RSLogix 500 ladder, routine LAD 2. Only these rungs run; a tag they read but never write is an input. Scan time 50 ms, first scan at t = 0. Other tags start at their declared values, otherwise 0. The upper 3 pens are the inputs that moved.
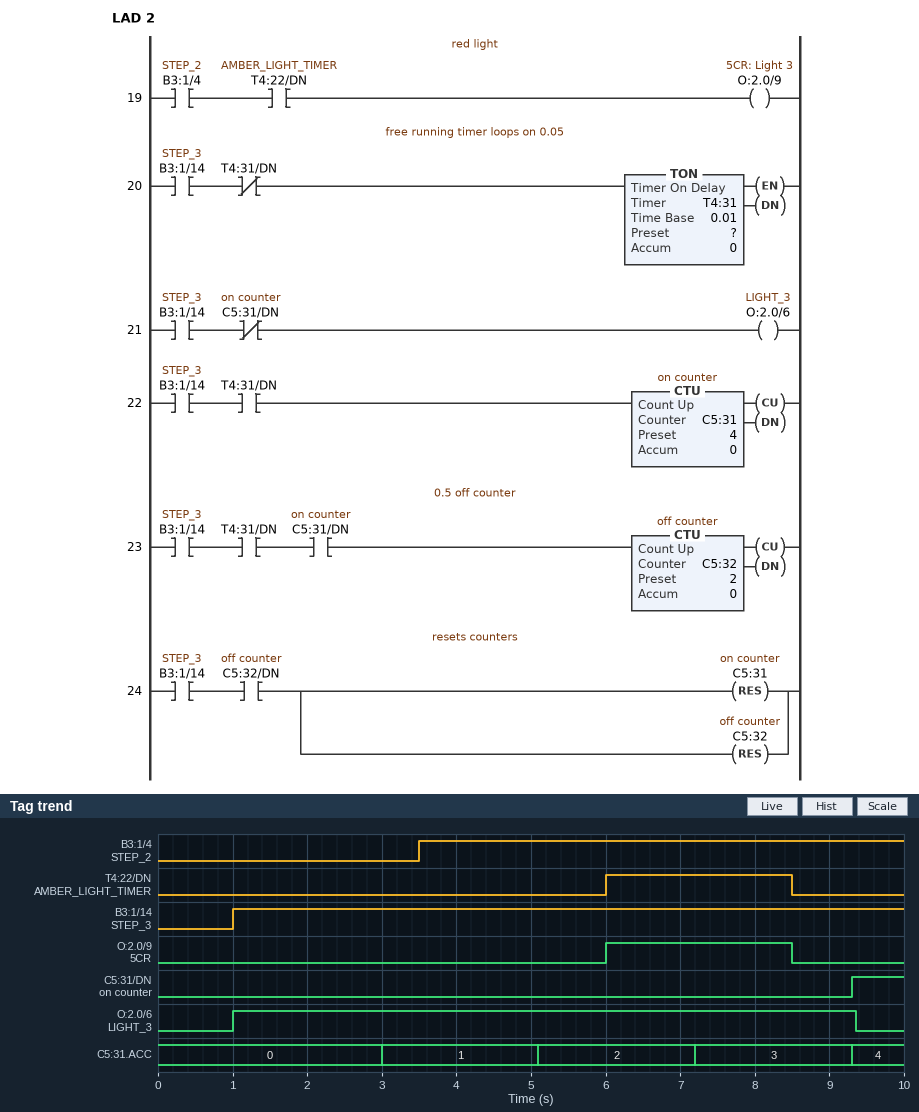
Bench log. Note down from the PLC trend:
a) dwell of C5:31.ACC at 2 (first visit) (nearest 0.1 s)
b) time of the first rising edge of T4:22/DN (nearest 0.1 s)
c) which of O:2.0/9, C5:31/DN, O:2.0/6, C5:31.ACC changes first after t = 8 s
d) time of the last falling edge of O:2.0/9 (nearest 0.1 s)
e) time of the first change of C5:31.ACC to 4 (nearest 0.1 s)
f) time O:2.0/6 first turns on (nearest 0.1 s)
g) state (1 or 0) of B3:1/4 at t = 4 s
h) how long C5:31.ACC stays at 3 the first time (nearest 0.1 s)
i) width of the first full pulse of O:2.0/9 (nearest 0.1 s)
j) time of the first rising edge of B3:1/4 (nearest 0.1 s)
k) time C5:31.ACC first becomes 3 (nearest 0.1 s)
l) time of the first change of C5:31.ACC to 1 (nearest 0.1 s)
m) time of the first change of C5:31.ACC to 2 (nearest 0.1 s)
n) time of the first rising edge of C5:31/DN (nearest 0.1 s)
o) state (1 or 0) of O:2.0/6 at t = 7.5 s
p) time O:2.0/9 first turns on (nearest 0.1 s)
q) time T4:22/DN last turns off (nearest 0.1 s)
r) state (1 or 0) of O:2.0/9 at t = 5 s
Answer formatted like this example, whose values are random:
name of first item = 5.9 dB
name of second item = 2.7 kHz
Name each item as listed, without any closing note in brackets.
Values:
dwell of C5:31.ACC at 2 (first visit) = 2.1 s
time of the first rising edge of T4:22/DN = 6.0 s
which of O:2.0/9, C5:31/DN, O:2.0/6, C5:31.ACC changes first after t = 8 s = O:2.0/9
time of the last falling edge of O:2.0/9 = 8.5 s
time of the first change of C5:31.ACC to 4 = 9.3 s
time O:2.0/6 first turns on = 1.0 s
state (1 or 0) of B3:1/4 at t = 4 s = 1
how long C5:31.ACC stays at 3 the first time = 2.1 s
width of the first full pulse of O:2.0/9 = 2.5 s
time of the first rising edge of B3:1/4 = 3.5 s
time C5:31.ACC first becomes 3 = 7.2 s
time of the first change of C5:31.ACC to 1 = 3.0 s
time of the first change of C5:31.ACC to 2 = 5.1 s
time of the first rising edge of C5:31/DN = 9.3 s
state (1 or 0) of O:2.0/6 at t = 7.5 s = 1
time O:2.0/9 first turns on = 6.0 s
time T4:22/DN last turns off = 8.5 s
state (1 or 0) of O:2.0/9 at t = 5 s = 0
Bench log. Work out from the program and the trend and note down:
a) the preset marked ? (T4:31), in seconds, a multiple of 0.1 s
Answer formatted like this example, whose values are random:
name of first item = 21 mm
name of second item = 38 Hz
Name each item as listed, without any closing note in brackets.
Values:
the preset marked ? (T4:31), in seconds, a multiple of 0.1 s = 2.0 s
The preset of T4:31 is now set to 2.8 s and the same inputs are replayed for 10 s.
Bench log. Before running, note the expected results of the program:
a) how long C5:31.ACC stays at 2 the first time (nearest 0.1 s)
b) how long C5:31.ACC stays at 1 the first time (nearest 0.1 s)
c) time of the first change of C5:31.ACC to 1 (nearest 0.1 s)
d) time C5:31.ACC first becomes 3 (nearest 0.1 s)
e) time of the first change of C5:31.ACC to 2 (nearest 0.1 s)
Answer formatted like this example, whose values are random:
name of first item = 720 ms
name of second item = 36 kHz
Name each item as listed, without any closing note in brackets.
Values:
how long C5:31.ACC stays at 2 the first time = 2.9 s
how long C5:31.ACC stays at 1 the first time = 2.9 s
time of the first change of C5:31.ACC to 1 = 3.8 s
time C5:31.ACC first becomes 3 = 9.6 s
time of the first change of C5:31.ACC to 2 = 6.7 s
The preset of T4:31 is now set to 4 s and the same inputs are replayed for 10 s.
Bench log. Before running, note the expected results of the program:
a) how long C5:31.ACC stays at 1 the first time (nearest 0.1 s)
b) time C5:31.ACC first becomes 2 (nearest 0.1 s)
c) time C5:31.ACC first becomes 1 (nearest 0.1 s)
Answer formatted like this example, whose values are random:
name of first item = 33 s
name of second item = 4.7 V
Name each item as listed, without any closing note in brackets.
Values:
how long C5:31.ACC stays at 1 the first time = 4.1 s
time C5:31.ACC first becomes 2 = 9.1 s
time C5:31.ACC first becomes 1 = 5.0 s
